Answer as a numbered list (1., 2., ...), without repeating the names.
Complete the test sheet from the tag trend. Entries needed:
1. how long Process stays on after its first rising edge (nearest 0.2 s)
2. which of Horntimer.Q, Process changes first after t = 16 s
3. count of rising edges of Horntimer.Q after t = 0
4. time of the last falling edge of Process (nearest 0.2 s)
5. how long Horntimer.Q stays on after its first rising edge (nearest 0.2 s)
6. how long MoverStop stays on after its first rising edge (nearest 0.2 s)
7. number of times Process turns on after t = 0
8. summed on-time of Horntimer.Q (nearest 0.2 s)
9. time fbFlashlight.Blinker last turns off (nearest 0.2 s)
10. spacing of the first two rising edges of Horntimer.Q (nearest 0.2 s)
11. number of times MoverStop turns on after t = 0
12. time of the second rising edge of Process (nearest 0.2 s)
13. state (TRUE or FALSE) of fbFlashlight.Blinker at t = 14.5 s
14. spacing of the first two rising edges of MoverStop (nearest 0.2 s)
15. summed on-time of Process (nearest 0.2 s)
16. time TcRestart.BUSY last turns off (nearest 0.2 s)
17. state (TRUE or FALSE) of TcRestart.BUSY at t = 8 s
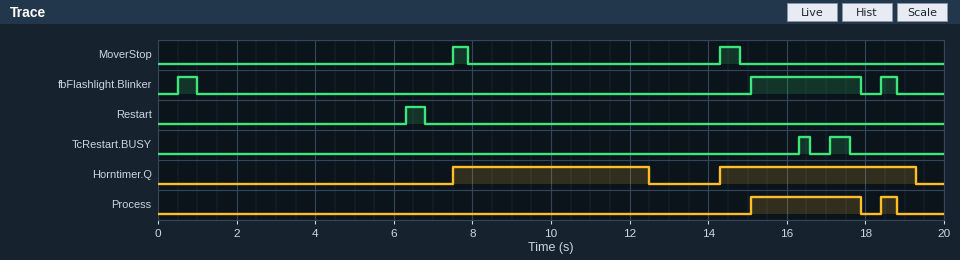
1. 2.8 s
2. Process
3. 2
4. 18.8 s
5. 5.0 s
6. 0.4 s
7. 2
8. 10.0 s
9. 18.8 s
10. 6.8 s
11. 2
12. 18.4 s
13. FALSE
14. 6.8 s
15. 3.2 s
16. 17.6 s
17. FALSE
